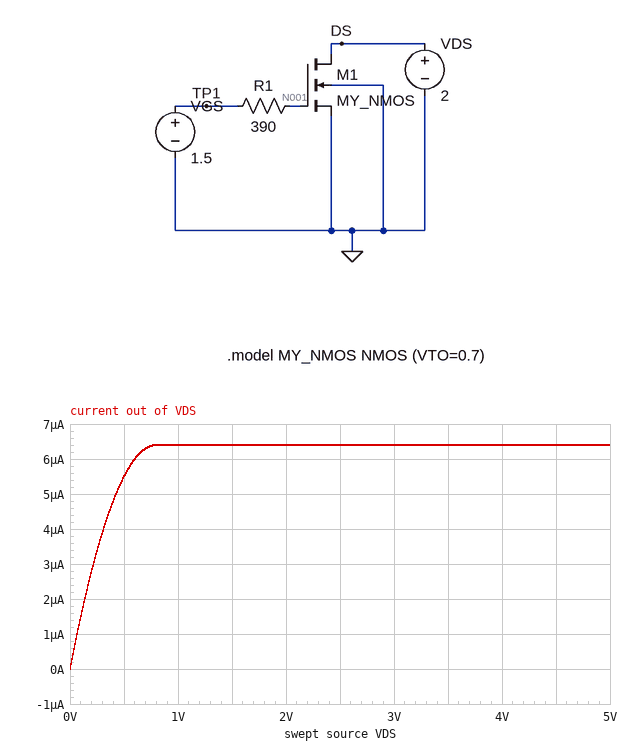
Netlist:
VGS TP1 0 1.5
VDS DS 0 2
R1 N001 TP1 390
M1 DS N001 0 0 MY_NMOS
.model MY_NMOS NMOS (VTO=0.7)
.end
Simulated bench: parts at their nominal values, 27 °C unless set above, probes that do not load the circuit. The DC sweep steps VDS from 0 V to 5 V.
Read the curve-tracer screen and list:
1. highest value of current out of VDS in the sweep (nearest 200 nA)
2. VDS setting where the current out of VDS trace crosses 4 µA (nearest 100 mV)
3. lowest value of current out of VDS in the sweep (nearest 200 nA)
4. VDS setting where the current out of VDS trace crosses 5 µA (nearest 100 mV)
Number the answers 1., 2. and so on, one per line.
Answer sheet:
1. 6.4 µA
2. 300 mV
3. 0 A
4. 400 mV
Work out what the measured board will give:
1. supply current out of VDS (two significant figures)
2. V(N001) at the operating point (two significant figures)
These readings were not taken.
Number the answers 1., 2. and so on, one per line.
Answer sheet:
1. 6.4 µA
2. 1.5 V
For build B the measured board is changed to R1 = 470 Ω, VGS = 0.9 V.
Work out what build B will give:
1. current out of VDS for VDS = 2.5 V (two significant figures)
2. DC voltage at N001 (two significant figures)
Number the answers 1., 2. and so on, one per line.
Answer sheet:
1. 400 nA
2. 900 mV
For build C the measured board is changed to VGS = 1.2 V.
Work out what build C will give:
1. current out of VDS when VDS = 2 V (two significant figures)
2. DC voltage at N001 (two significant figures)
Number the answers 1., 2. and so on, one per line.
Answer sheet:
1. 2.5 µA
2. 1.2 V
